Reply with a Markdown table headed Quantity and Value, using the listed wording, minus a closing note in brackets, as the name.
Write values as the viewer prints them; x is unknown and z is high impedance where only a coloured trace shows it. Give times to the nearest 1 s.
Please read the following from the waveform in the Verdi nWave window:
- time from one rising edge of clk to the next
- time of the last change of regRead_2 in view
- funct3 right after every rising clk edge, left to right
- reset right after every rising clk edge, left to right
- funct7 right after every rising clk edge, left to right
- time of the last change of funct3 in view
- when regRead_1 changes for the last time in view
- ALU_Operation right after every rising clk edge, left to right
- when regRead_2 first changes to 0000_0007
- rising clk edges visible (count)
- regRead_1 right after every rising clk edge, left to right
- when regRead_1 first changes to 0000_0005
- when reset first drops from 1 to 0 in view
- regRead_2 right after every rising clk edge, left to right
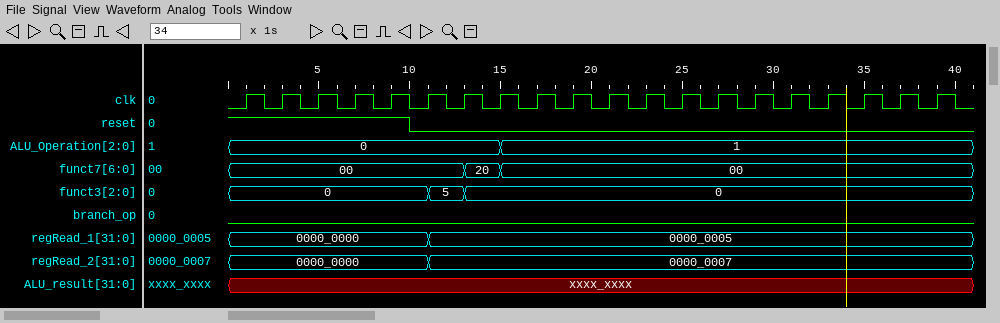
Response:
| Quantity | Value |
|---|---|
| time from one rising edge of clk to the next | 2 s |
| time of the last change of regRead_2 in view | 11 s |
| funct3 right after every rising clk edge, left to right | 0, 0, 0, 0, 0, 5, 0, 0, 0, 0, 0, 0, 0, 0, 0, 0, 0, 0, 0, 0 |
| reset right after every rising clk edge, left to right | 1 1 1 1 1 0 0 0 0 0 0 0 0 0 0 0 0 0 0 0 |
| funct7 right after every rising clk edge, left to right | 00, 00, 00, 00, 00, 00, 20, 00, 00, 00, 00, 00, 00, 00, 00, 00, 00, 00, 00, 00 |
| time of the last change of funct3 in view | 13 s |
| when regRead_1 changes for the last time in view | 11 s |
| ALU_Operation right after every rising clk edge, left to right | 0, 0, 0, 0, 0, 0, 0, 1, 1, 1, 1, 1, 1, 1, 1, 1, 1, 1, 1, 1 |
| when regRead_2 first changes to 0000_0007 | 11 s |
| rising clk edges visible | 20 |
| regRead_1 right after every rising clk edge, left to right | 0000_0000, 0000_0000, 0000_0000, 0000_0000, 0000_0000, 0000_0005, 0000_0005, 0000_0005, 0000_0005, 0000_0005, 0000_0005, 0000_0005, 0000_0005, 0000_0005, 0000_0005, 0000_0005, 0000_0005, 0000_0005, 0000_0005, 0000_0005 |
| when regRead_1 first changes to 0000_0005 | 11 s |
| when reset first drops from 1 to 0 in view | 10 s |
| regRead_2 right after every rising clk edge, left to right | 0000_0000, 0000_0000, 0000_0000, 0000_0000, 0000_0000, 0000_0007, 0000_0007, 0000_0007, 0000_0007, 0000_0007, 0000_0007, 0000_0007, 0000_0007, 0000_0007, 0000_0007, 0000_0007, 0000_0007, 0000_0007, 0000_0007, 0000_0007 |
